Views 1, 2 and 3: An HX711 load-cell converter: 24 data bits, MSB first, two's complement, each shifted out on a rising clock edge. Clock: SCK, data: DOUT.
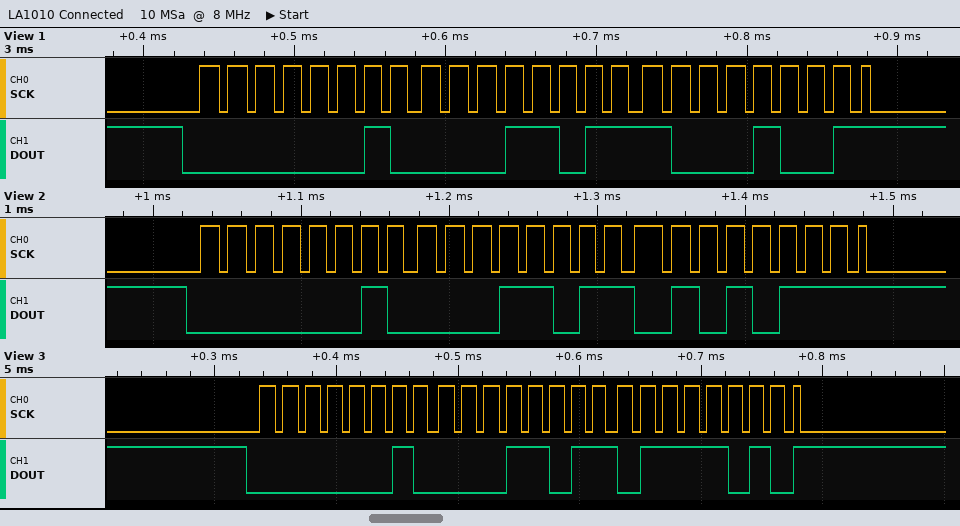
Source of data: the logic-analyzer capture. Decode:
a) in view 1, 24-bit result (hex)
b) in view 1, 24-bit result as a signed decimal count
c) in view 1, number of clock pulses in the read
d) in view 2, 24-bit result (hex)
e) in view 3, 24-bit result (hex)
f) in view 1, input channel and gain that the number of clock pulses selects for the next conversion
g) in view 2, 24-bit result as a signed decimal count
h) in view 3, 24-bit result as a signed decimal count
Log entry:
0x021B89
138121
25
0x021B57
0x021B7A
channel A, gain 128
138071
138106
